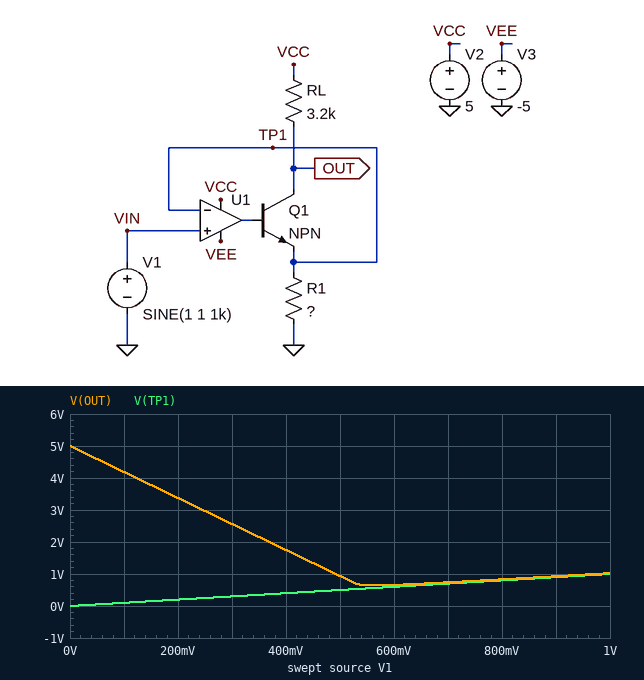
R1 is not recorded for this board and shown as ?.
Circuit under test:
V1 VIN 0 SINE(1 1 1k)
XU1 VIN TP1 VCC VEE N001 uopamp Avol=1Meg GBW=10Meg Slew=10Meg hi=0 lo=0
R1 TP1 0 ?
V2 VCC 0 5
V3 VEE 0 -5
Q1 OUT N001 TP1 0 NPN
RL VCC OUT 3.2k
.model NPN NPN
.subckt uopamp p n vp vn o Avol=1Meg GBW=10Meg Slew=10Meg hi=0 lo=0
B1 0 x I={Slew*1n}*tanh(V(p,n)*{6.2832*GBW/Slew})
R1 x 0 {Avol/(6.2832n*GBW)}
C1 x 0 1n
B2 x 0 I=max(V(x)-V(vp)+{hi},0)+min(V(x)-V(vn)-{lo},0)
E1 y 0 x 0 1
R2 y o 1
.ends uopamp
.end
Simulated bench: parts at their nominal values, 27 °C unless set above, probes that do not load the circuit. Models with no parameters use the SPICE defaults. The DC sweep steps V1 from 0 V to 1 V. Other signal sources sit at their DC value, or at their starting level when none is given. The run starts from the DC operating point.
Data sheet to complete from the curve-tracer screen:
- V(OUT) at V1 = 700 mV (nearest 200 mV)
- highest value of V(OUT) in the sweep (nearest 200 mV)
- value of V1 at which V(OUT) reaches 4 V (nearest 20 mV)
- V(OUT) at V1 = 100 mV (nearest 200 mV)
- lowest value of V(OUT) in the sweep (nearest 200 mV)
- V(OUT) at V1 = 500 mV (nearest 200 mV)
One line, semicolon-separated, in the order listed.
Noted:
800 mV; 5.0 V; 120 mV; 4.2 V; 600 mV; 1.0 V
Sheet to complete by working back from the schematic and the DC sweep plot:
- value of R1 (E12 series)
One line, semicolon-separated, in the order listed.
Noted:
390 Ω
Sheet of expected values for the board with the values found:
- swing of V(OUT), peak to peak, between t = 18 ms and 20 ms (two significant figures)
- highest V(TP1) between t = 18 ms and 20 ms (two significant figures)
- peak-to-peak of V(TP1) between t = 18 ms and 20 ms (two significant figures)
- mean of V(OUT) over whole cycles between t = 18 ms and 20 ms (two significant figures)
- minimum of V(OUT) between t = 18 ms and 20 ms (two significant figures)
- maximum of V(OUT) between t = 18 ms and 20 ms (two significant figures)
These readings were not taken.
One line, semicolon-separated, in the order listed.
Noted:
4.4 V; 2.0 V; 2.0 V; 2.2 V; 640 mV; 5.0 V
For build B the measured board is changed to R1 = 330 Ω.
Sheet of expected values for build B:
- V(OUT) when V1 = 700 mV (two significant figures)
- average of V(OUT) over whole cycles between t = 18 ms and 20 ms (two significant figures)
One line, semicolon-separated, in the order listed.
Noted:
730 mV; 2.1 V
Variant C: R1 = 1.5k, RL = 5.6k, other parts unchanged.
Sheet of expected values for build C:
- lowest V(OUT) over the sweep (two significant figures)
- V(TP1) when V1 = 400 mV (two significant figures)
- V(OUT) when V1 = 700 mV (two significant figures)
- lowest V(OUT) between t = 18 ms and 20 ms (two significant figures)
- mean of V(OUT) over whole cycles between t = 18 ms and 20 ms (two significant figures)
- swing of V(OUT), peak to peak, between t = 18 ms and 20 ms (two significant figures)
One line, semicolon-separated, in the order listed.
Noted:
1.3 V; 400 mV; 2.4 V; 1.2 V; 2.7 V; 3.8 V
